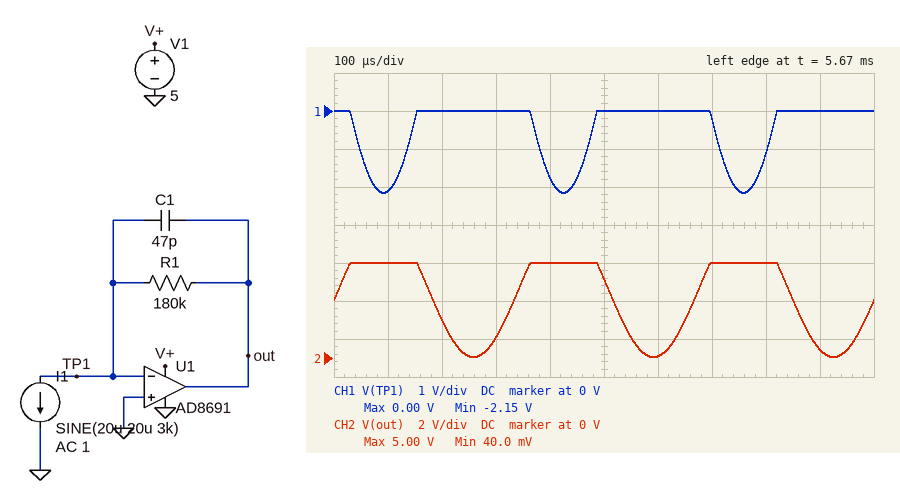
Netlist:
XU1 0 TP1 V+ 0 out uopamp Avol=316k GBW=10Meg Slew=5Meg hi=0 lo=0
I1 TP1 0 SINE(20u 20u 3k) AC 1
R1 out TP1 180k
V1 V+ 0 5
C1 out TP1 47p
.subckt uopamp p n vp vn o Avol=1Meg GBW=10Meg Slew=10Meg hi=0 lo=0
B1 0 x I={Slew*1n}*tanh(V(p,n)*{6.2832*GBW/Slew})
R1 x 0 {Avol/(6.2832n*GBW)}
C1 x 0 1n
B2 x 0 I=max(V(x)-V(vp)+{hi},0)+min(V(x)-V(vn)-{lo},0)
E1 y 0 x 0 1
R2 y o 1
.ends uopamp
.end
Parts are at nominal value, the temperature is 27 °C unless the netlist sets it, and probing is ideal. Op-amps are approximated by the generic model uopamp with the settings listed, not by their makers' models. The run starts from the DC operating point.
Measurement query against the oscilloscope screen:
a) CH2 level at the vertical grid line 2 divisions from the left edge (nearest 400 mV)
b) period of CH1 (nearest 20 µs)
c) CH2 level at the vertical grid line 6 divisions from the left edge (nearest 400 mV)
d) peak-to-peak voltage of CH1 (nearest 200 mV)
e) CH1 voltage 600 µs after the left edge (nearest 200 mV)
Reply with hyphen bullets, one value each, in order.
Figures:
- 2.0 V
- 340 µs
- 0 V
- 2.2 V
- 0 V
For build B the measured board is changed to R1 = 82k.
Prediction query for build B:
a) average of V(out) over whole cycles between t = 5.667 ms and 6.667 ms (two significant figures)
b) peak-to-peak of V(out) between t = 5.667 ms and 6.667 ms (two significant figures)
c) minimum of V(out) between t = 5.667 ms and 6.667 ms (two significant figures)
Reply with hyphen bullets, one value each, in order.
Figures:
- 1.6 V
- 3.3 V
- 4.3 mV
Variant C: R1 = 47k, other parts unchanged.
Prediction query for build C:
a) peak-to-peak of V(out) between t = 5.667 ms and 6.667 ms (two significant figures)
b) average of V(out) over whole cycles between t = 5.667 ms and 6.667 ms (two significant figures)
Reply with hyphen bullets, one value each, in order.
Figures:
- 1.9 V
- 940 mV
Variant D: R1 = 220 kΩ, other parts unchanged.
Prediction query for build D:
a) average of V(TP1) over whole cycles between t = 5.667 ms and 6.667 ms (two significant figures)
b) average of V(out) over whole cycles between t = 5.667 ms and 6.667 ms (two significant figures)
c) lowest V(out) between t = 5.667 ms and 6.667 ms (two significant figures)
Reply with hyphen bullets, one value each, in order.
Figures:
- -1.1 V
- 3.3 V
- 81 mV
